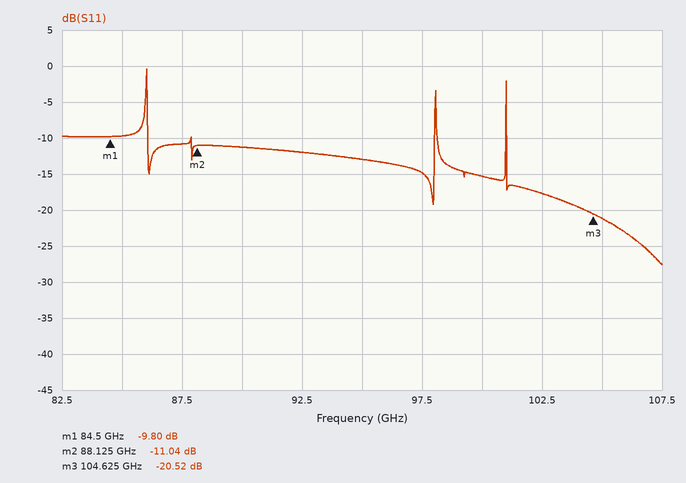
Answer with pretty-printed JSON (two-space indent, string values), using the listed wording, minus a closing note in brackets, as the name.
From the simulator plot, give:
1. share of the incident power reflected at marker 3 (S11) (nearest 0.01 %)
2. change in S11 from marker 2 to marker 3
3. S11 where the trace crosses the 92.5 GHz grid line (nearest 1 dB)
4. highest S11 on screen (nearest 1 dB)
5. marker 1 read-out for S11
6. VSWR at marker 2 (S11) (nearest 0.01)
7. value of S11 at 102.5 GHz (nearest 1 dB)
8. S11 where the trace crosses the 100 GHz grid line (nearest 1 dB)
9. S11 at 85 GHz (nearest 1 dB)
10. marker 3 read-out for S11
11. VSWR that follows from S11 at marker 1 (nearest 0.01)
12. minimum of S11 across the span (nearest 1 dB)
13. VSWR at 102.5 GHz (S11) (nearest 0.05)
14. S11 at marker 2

{
  "share of the incident power reflected at marker 3 (S11)": "0.89 %",
  "change in S11 from marker 2 to marker 3": "-9.48 dB",
  "S11 where the trace crosses the 92.5 GHz grid line": "-12 dB",
  "highest S11 on screen": "0 dB",
  "marker 1 read-out for S11": "-9.80 dB",
  "VSWR at marker 2 (S11)": "1.78",
  "value of S11 at 102.5 GHz": "-18 dB",
  "S11 where the trace crosses the 100 GHz grid line": "-15 dB",
  "S11 at 85 GHz": "-10 dB",
  "marker 3 read-out for S11": "-20.52 dB",
  "VSWR that follows from S11 at marker 1": "1.96",
  "minimum of S11 across the span": "-28 dB",
  "VSWR at 102.5 GHz (S11)": "1.30",
  "S11 at marker 2": "-11.04 dB"
}
